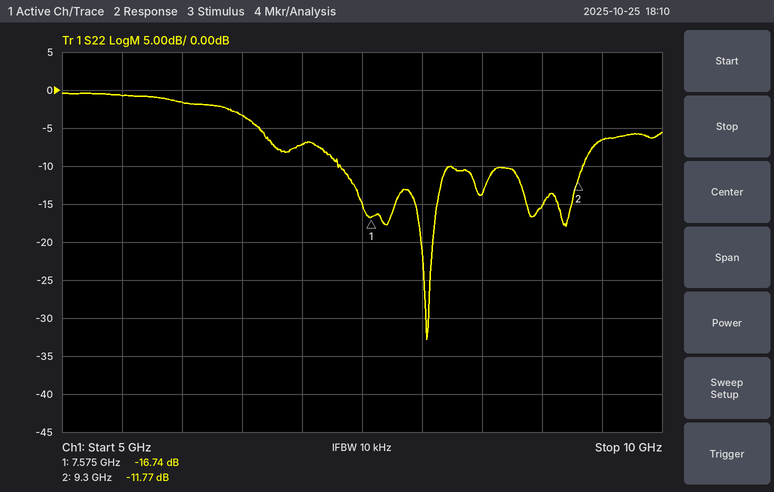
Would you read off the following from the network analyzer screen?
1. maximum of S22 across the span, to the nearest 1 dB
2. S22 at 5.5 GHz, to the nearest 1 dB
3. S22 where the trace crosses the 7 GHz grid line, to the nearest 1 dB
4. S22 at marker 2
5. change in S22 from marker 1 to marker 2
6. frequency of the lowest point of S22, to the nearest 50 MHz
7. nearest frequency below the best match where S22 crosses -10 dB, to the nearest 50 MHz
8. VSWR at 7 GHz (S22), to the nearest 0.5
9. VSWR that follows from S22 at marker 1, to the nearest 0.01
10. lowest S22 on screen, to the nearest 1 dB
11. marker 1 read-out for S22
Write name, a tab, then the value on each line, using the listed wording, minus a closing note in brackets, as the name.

maximum of S22 across the span, to the nearest 1 dB	0 dB
S22 at 5.5 GHz, to the nearest 1 dB	-1 dB
S22 where the trace crosses the 7 GHz grid line, to the nearest 1 dB	-7 dB
S22 at marker 2	-11.77 dB
change in S22 from marker 1 to marker 2	4.97 dB
frequency of the lowest point of S22, to the nearest 50 MHz	8.05 GHz
nearest frequency below the best match where S22 crosses -10 dB, to the nearest 50 MHz	7.30 GHz
VSWR at 7 GHz (S22), to the nearest 0.5	2.5
VSWR that follows from S22 at marker 1, to the nearest 0.01	1.34
lowest S22 on screen, to the nearest 1 dB	-33 dB
marker 1 read-out for S22	-16.74 dB
